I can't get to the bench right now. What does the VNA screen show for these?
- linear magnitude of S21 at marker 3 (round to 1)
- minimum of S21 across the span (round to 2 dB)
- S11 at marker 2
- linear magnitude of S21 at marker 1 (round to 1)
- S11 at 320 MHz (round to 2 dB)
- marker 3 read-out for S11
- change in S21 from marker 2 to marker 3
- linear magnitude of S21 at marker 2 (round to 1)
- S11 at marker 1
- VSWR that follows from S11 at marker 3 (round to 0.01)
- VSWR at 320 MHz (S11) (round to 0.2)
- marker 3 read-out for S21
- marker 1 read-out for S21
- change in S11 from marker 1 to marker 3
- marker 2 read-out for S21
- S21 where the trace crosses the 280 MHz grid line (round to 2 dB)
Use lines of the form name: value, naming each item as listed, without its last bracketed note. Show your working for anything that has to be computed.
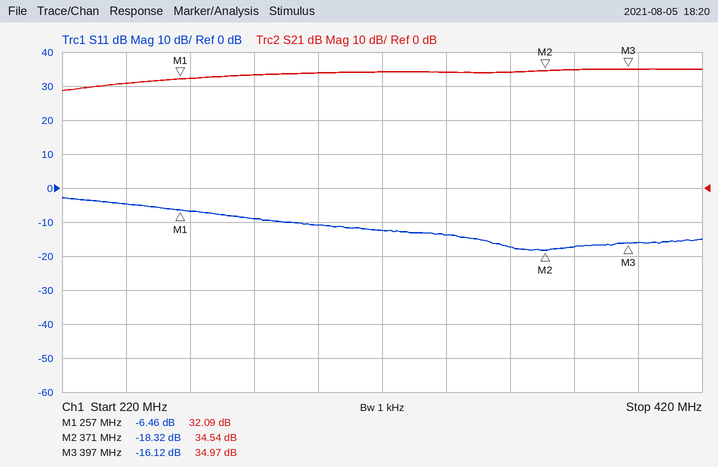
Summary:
linear magnitude of S21 at marker 3: 10^(34.97/20) ≈ 56
minimum of S21 across the span: 28 dB
S11 at marker 2: -18.32 dB
linear magnitude of S21 at marker 1: 10^(32.09/20) ≈ 40
S11 at 320 MHz: -12 dB
marker 3 read-out for S11: -16.12 dB
change in S21 from marker 2 to marker 3: 34.97 − (34.54) = 0.43 dB
linear magnitude of S21 at marker 2: 10^(34.54/20) ≈ 53
S11 at marker 1: -6.46 dB
VSWR that follows from S11 at marker 3: (1 + 0.1563)/(1 − 0.1563) ≈ 1.37
VSWR at 320 MHz (S11): |Γ| = 10^(-12/20) = 0.2512; VSWR = (1 + 0.2512)/(1 − 0.2512) ≈ 1.67, so 1.6 to the nearest 0.2
marker 3 read-out for S21: 34.97 dB
marker 1 read-out for S21: 32.09 dB
change in S11 from marker 1 to marker 3: -16.12 − (-6.46) = -9.66 dB
marker 2 read-out for S21: 34.54 dB
S21 where the trace crosses the 280 MHz grid line: 34 dB
